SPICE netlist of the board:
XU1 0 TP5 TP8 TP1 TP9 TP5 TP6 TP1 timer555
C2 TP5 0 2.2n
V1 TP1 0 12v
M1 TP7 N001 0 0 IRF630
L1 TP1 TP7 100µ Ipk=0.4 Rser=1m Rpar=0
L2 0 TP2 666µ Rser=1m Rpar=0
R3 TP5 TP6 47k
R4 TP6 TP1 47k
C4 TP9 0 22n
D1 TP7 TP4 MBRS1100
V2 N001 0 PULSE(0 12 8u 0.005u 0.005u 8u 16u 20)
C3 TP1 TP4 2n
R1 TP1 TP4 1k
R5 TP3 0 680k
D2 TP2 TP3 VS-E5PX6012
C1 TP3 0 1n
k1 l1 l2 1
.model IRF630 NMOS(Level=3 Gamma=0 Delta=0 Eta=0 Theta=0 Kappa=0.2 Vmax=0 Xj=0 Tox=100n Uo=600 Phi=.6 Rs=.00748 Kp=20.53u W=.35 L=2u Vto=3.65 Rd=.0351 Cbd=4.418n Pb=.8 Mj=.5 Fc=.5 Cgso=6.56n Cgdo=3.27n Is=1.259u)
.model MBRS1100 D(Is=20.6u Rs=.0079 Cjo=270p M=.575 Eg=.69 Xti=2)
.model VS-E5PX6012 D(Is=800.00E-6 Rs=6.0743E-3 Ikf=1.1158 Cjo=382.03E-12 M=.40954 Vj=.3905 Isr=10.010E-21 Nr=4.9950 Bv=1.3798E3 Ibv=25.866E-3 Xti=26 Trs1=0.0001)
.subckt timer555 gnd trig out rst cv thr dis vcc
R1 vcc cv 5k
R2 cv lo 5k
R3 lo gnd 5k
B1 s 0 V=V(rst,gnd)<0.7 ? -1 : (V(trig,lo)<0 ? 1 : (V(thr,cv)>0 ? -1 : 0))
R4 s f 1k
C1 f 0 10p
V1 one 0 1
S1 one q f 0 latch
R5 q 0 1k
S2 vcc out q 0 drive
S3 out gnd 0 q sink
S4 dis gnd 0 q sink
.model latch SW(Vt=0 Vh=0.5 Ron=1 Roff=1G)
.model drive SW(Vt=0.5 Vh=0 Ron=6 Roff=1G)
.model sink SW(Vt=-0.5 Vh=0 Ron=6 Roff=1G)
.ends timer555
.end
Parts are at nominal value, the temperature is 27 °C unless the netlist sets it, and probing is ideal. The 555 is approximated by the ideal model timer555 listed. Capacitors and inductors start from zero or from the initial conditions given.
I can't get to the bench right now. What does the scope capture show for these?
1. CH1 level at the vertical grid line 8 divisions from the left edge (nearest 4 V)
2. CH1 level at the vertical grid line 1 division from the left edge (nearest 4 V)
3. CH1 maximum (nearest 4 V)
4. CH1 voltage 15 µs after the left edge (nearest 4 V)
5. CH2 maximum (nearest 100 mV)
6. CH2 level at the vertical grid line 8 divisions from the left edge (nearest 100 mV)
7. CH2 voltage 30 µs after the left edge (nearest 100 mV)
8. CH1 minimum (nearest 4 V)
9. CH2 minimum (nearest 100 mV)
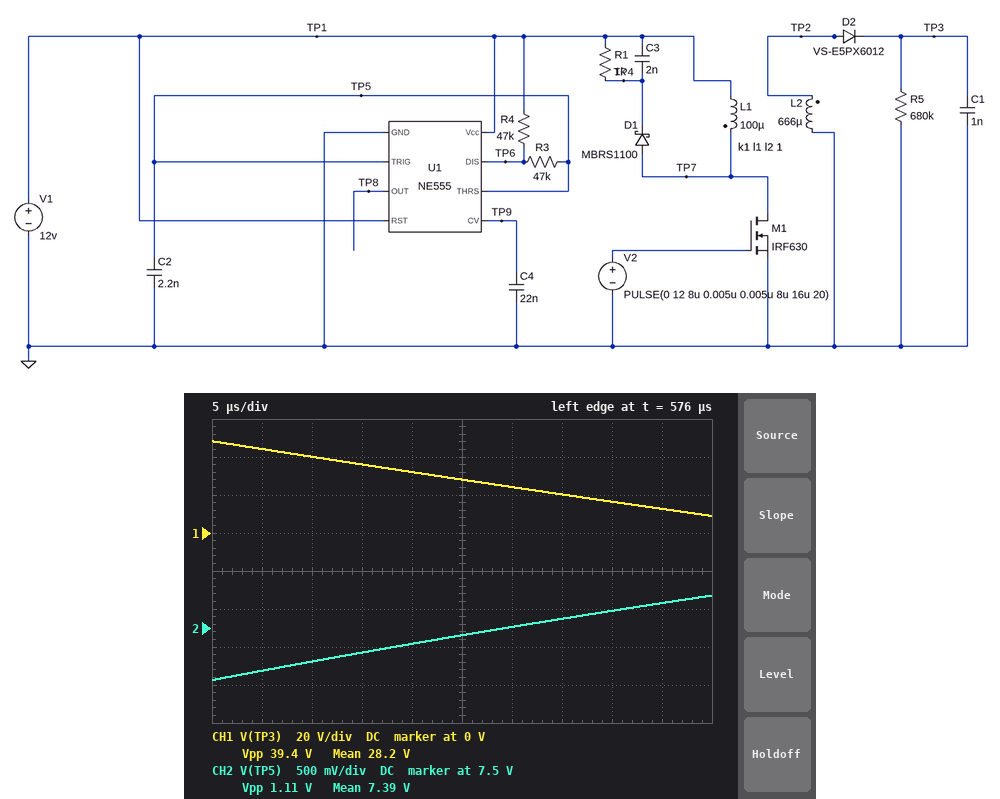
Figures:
16 V
44 V
48 V
36 V
7.9 V
7.7 V
7.5 V
8 V
6.8 V
